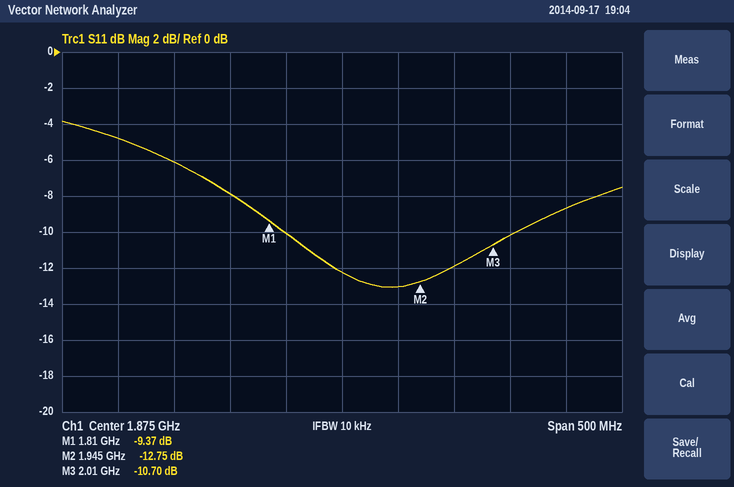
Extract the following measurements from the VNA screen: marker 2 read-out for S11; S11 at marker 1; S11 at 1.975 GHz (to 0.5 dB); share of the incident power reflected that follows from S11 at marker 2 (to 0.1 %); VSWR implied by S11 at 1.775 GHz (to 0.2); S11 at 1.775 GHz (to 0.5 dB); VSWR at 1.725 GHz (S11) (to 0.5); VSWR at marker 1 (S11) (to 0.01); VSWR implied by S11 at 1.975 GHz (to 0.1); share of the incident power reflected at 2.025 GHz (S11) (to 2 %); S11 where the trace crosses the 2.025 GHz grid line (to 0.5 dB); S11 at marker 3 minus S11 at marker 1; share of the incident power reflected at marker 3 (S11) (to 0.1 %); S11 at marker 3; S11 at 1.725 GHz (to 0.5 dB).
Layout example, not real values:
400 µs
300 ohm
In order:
-12.75 dB
-9.37 dB
-12.0 dB
5.3 %
2.4
-8.0 dB
3.0
2.03
1.7
10 %
-10.0 dB
-1.33 dB
8.5 %
-10.70 dB
-6.0 dB
